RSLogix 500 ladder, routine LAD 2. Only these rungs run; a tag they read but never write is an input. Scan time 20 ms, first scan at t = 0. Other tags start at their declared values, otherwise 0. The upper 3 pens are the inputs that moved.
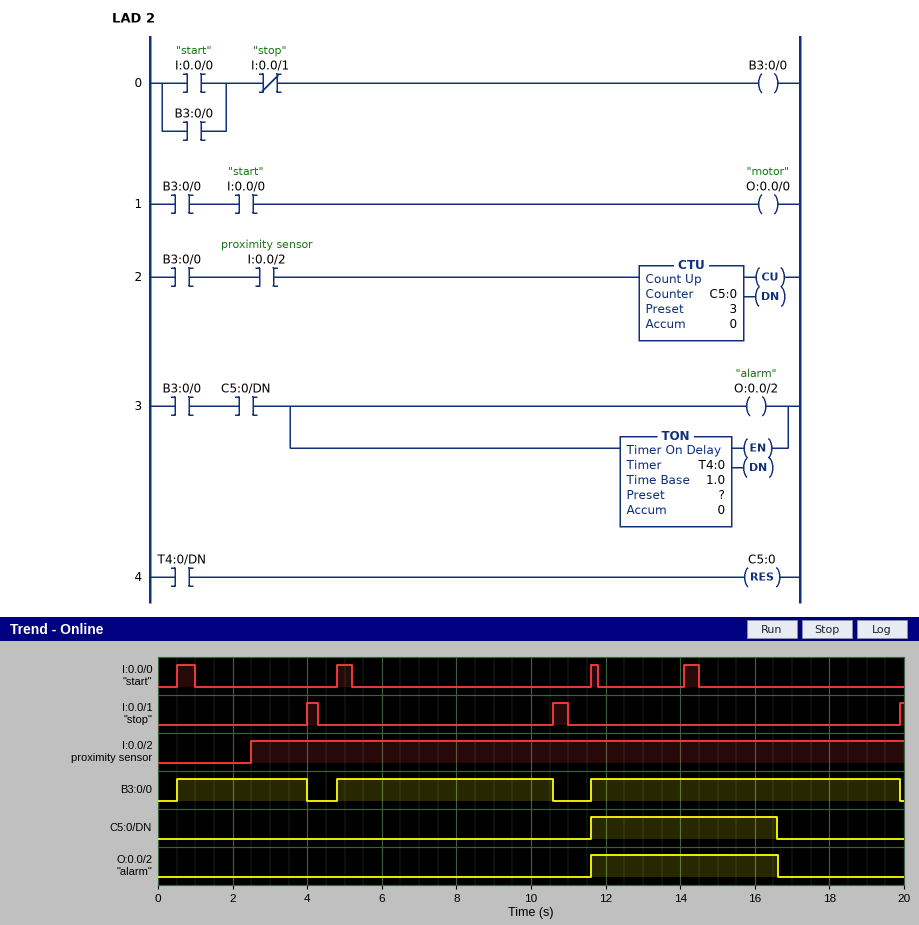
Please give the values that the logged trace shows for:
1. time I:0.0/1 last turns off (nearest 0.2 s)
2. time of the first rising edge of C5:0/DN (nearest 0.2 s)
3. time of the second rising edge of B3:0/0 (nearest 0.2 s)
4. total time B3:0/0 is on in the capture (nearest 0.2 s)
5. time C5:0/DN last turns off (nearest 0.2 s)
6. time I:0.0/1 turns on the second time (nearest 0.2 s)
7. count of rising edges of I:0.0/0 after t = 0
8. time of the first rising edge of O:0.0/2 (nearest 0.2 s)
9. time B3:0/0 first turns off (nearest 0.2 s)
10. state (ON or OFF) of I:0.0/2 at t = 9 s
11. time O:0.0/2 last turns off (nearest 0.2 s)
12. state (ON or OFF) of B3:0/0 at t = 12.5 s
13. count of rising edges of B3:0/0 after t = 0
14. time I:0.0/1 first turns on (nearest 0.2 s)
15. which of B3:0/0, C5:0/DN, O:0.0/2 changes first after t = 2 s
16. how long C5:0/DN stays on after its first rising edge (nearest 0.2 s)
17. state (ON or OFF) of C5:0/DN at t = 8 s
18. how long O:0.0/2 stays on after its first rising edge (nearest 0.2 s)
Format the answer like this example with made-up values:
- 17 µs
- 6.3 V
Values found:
- 11.0 s
- 11.6 s
- 4.8 s
- 17.6 s
- 16.6 s
- 10.6 s
- 4
- 11.6 s
- 4.0 s
- ON
- 16.6 s
- ON
- 3
- 4.0 s
- B3:0/0
- 5.0 s
- OFF
- 5.0 s
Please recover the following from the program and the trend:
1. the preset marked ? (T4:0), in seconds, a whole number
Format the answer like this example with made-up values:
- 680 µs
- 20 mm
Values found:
- 5 s
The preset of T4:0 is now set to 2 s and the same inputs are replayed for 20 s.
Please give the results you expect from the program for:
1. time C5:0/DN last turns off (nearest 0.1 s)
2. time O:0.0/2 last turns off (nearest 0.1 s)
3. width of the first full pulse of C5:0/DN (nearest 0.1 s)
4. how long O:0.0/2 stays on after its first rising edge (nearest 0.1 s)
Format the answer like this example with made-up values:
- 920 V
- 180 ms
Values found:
- 13.6 s
- 13.6 s
- 2.0 s
- 2.0 s
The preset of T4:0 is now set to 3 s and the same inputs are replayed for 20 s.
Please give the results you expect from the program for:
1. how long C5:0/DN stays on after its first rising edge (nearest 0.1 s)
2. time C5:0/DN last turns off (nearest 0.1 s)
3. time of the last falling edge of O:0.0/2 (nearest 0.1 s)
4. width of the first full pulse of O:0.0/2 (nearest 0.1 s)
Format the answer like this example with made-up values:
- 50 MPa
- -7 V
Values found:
- 3.0 s
- 14.6 s
- 14.6 s
- 3.0 s
